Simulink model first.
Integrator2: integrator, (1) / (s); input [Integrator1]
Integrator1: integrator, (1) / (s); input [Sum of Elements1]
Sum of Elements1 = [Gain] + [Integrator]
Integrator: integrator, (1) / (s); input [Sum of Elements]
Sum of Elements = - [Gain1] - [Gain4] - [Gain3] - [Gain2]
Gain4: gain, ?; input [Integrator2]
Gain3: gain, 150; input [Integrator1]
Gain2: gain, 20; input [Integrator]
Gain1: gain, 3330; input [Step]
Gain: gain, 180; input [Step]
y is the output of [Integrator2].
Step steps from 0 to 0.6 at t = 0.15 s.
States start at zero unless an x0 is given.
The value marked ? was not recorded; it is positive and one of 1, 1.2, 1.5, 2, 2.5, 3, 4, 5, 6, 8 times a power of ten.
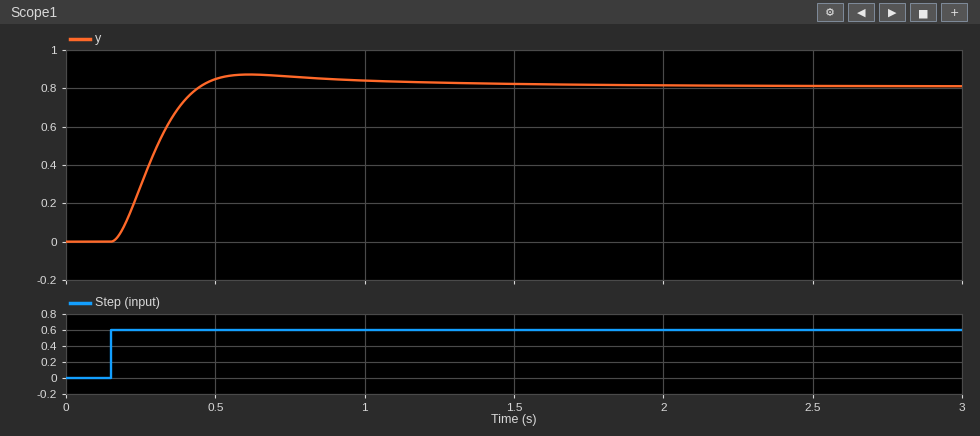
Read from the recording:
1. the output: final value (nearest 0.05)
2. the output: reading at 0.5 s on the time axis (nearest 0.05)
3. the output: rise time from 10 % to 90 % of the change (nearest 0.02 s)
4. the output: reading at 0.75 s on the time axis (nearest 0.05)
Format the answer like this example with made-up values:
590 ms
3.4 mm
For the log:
0.80
0.85
0.20 s
0.85
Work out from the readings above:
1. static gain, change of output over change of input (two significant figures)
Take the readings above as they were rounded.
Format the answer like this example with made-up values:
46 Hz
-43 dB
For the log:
1.3
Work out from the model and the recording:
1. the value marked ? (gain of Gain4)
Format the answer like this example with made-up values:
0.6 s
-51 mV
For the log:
200
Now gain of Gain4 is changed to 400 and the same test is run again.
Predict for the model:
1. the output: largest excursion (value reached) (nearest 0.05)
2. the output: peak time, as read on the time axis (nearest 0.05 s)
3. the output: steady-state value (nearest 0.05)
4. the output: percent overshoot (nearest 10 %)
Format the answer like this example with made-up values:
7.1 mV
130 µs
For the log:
0.75
0.50 s
0.40
90 %
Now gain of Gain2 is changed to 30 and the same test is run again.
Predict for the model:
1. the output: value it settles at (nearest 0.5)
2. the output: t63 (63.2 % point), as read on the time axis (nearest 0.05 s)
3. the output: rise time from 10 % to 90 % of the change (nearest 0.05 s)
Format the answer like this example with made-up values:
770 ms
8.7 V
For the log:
6.0
0.85 s
1.20 s
